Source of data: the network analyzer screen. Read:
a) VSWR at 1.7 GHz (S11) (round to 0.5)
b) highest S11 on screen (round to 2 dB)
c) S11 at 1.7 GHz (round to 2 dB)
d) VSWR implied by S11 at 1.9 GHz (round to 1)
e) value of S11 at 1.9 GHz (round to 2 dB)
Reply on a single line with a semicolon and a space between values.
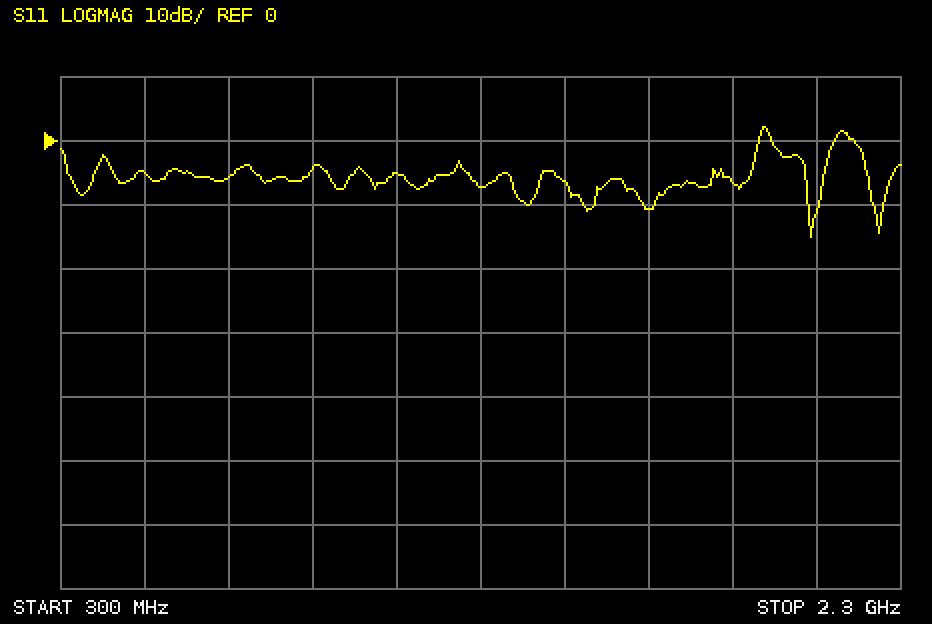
2.0; 2 dB; -10 dB; 3; -6 dB
